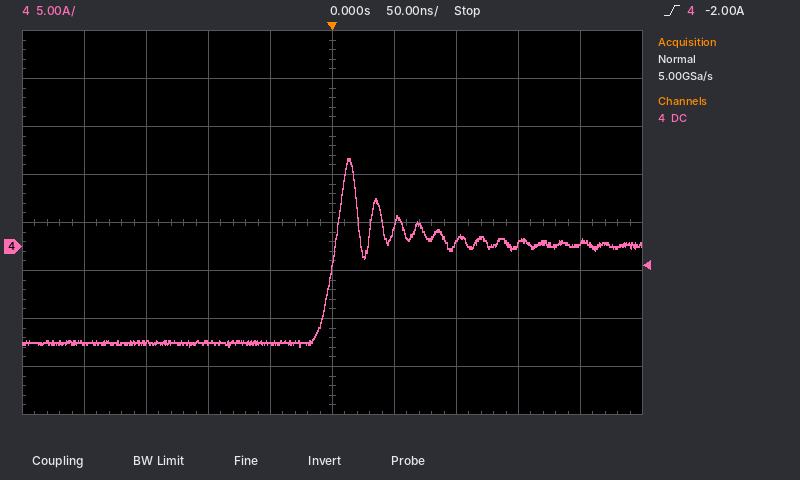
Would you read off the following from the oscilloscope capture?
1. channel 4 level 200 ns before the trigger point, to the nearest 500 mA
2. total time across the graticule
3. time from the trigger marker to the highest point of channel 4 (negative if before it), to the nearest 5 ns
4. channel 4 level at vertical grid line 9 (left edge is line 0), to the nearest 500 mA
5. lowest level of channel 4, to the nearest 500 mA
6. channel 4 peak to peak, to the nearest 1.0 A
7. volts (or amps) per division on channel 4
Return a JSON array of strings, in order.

["-10.0 A", "500 ns", "+15 ns", "500 mA", "-10.5 A", "20.0 A", "5 A"]
